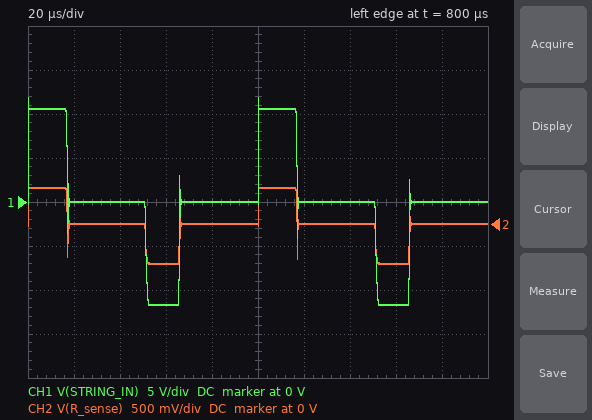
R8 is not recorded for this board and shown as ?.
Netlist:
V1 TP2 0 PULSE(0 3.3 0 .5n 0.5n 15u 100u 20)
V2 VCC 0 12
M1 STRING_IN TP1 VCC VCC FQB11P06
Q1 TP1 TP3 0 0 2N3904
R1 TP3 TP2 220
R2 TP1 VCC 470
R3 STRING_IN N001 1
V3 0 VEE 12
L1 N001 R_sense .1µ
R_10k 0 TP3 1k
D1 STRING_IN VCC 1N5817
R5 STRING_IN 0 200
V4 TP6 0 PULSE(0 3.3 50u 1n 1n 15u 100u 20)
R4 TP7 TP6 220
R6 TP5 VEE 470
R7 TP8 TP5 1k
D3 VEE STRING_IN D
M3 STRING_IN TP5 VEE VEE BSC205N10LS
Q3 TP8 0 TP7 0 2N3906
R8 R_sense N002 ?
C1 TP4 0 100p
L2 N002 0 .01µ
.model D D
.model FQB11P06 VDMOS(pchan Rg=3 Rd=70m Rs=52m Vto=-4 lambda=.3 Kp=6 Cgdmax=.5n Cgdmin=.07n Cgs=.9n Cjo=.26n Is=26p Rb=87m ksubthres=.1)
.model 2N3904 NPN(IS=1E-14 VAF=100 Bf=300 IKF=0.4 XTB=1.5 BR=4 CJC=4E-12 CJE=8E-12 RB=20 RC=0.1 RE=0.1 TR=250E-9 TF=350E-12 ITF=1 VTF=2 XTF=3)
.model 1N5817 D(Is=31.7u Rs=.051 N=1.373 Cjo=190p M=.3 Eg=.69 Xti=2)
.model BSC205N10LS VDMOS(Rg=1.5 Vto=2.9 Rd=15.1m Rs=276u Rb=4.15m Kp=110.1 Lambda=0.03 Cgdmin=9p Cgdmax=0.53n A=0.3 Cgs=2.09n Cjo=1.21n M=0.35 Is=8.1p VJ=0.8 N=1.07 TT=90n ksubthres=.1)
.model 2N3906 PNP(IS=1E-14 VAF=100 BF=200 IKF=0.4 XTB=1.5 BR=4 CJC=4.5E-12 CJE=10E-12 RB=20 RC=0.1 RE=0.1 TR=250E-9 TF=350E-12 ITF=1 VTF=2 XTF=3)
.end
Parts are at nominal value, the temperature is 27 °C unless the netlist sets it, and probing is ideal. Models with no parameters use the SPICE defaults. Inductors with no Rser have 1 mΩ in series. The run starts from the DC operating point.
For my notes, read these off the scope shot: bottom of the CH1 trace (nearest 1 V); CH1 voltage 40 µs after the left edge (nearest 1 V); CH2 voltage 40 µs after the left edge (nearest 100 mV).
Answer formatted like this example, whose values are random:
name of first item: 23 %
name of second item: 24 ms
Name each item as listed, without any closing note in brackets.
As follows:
bottom of the CH1 trace: -12 V
CH1 voltage 40 µs after the left edge: 0 V
CH2 voltage 40 µs after the left edge: 0 V
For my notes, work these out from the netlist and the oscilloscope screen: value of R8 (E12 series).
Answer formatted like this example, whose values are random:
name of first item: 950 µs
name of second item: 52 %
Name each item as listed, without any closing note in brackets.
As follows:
value of R8: 0.039 Ω
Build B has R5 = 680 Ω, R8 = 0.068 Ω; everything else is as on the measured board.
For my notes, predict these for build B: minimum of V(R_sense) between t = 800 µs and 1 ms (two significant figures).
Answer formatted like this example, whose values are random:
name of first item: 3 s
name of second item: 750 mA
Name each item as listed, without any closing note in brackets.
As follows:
minimum of V(R_sense) between t = 800 µs and 1 ms: -760 mV
